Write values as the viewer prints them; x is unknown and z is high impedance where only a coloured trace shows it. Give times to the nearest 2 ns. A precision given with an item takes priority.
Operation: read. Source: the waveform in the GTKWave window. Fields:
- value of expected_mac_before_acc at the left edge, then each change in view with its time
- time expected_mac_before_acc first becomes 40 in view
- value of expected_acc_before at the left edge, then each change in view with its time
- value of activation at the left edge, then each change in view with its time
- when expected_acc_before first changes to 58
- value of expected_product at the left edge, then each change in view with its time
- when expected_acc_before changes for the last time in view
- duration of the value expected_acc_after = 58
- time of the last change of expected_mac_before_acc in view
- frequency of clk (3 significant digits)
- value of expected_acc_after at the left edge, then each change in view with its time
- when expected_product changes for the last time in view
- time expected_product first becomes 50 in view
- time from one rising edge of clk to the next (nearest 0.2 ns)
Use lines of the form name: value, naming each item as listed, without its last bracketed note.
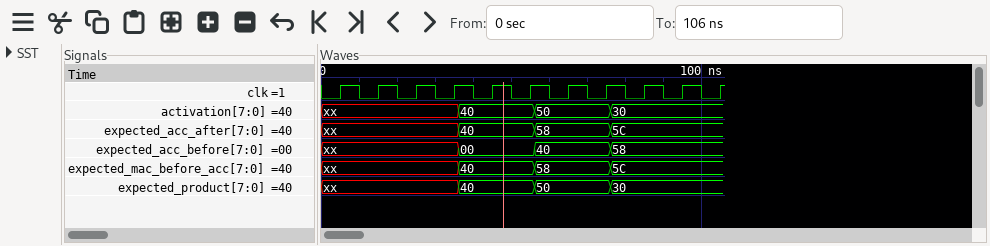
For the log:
value of expected_mac_before_acc at the left edge, then each change in view with its time: xx, 40 at 36 ns, 58 at 56 ns, 5C at 76 ns
time expected_mac_before_acc first becomes 40 in view: 36 ns
value of expected_acc_before at the left edge, then each change in view with its time: xx, 00 at 36 ns, 40 at 56 ns, 58 at 76 ns
value of activation at the left edge, then each change in view with its time: xx, 40 at 36 ns, 50 at 56 ns, 30 at 76 ns
when expected_acc_before first changes to 58: 76 ns
value of expected_product at the left edge, then each change in view with its time: xx, 40 at 36 ns, 50 at 56 ns, 30 at 76 ns
when expected_acc_before changes for the last time in view: 76 ns
duration of the value expected_acc_after = 58: 20 ns
time of the last change of expected_mac_before_acc in view: 76 ns
frequency of clk: 100 MHz
value of expected_acc_after at the left edge, then each change in view with its time: xx, 40 at 36 ns, 58 at 56 ns, 5C at 76 ns
when expected_product changes for the last time in view: 76 ns
time expected_product first becomes 50 in view: 56 ns
time from one rising edge of clk to the next: 10 ns
